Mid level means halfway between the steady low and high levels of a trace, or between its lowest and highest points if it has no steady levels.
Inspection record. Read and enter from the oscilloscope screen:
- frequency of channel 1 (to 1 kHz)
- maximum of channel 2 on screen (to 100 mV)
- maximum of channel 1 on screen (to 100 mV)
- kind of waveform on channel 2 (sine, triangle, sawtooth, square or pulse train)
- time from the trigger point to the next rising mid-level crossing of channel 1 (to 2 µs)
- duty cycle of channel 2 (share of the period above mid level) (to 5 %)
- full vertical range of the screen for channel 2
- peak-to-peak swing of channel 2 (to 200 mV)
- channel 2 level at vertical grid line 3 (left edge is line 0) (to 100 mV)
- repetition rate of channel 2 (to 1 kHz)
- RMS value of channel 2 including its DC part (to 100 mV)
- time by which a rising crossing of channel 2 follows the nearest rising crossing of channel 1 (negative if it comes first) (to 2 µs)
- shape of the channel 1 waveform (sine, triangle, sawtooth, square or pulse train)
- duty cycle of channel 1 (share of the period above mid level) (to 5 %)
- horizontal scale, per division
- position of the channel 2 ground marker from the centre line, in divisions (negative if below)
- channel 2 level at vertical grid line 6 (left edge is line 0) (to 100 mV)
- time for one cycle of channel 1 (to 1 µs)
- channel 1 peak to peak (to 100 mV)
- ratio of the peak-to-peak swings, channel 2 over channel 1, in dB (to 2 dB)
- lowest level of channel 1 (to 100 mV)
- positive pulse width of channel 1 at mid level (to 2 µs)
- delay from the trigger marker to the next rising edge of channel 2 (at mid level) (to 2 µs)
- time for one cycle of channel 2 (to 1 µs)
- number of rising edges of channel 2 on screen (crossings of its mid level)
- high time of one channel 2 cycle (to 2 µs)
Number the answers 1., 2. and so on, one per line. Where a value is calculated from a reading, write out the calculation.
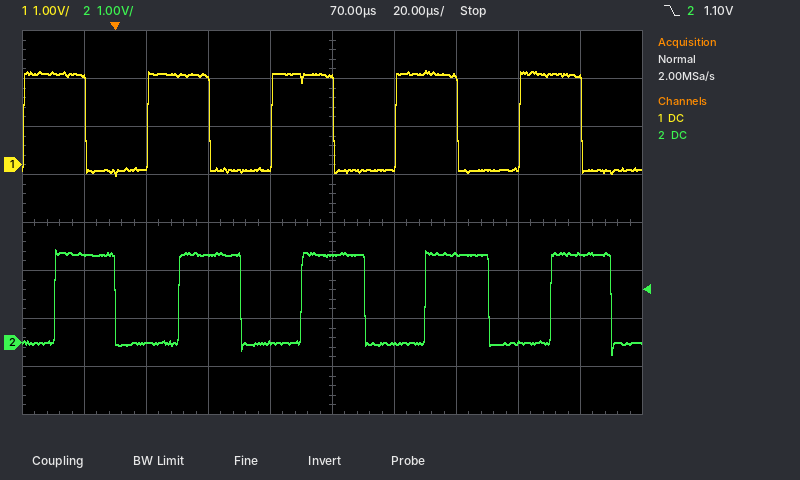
1. 1 / 40 µs ≈ 25 kHz
2. 1.9 V
3. 2.0 V
4. square
5. 10 µs
6. 20 µs / 40 µs ≈ 50 %
7. 8 V
8. 2.2 V
9. 1.8 V
10. 1 / 40 µs ≈ 25 kHz
11. √(0.5 × (1.9 V)² + 0.5 × (0.0 V)²) ≈ 1.3 V
12. +10 µs
13. square
14. 20 µs / 40 µs ≈ 50 %
15. 20 µs
16. -2.5 div
17. 0.0 V
18. 40 µs
19. 2.0 V − (-200 mV) = 2.2 V
20. 20 log10(2.2 V / 2.2 V) ≈ 0 dB
21. -200 mV
22. 20 µs
23. 20 µs
24. 40 µs
25. 5
26. 20 µs
